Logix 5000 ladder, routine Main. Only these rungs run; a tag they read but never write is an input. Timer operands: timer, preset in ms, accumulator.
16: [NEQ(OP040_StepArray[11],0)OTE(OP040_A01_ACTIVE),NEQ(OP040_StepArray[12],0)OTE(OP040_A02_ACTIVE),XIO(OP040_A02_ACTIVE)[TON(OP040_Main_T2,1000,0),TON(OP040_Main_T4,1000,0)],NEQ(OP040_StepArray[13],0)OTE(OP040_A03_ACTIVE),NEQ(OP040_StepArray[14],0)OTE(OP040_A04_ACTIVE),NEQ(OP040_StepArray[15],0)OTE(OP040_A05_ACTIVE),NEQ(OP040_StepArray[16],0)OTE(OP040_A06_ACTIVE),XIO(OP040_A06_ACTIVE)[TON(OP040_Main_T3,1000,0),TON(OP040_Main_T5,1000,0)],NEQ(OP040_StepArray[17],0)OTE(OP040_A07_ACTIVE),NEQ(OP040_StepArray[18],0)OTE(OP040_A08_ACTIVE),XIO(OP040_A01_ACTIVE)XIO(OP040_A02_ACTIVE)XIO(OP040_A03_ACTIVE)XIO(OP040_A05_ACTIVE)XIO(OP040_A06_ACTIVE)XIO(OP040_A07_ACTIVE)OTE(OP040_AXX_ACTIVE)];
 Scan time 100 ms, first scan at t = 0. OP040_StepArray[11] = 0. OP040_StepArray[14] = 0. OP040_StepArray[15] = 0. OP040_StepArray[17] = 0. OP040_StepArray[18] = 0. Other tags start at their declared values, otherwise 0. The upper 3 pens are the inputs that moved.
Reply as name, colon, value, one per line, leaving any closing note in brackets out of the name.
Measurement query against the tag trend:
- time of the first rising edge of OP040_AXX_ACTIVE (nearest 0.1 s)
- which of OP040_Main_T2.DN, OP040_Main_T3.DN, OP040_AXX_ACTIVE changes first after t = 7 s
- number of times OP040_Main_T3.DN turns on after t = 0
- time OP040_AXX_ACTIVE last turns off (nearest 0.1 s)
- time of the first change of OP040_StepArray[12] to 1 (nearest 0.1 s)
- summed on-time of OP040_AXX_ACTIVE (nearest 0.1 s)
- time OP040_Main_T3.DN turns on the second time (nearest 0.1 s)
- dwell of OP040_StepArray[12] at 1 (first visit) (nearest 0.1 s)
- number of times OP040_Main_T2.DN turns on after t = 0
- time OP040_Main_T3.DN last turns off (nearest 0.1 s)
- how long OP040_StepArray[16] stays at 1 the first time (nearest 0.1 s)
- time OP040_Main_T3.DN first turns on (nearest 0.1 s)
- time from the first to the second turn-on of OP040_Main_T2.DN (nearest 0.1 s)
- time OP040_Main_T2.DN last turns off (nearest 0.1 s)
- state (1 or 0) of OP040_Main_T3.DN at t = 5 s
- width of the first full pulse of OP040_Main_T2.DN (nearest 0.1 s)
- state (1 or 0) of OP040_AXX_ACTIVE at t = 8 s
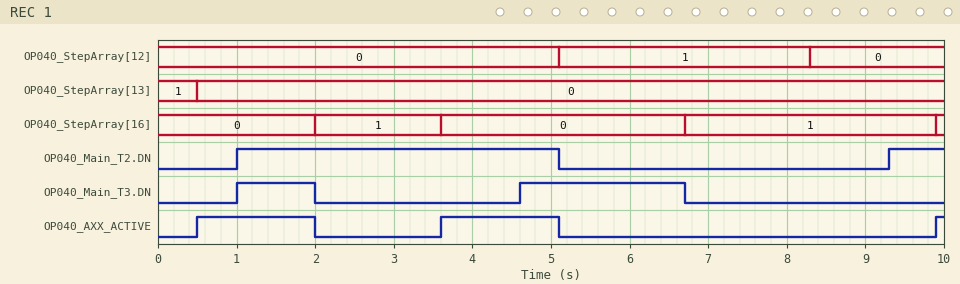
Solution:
time of the first rising edge of OP040_AXX_ACTIVE: 0.5 s
which of OP040_Main_T2.DN, OP040_Main_T3.DN, OP040_AXX_ACTIVE changes first after t = 7 s: OP040_Main_T2.DN
number of times OP040_Main_T3.DN turns on after t = 0: 2
time OP040_AXX_ACTIVE last turns off: 5.1 s
time of the first change of OP040_StepArray[12] to 1: 5.1 s
summed on-time of OP040_AXX_ACTIVE: 3.1 s
time OP040_Main_T3.DN turns on the second time: 4.6 s
dwell of OP040_StepArray[12] at 1 (first visit): 3.2 s
number of times OP040_Main_T2.DN turns on after t = 0: 2
time OP040_Main_T3.DN last turns off: 6.7 s
how long OP040_StepArray[16] stays at 1 the first time: 1.6 s
time OP040_Main_T3.DN first turns on: 1.0 s
time from the first to the second turn-on of OP040_Main_T2.DN: 8.3 s
time OP040_Main_T2.DN last turns off: 5.1 s
state (1 or 0) of OP040_Main_T3.DN at t = 5 s: 1
width of the first full pulse of OP040_Main_T2.DN: 4.1 s
state (1 or 0) of OP040_AXX_ACTIVE at t = 8 s: 0
